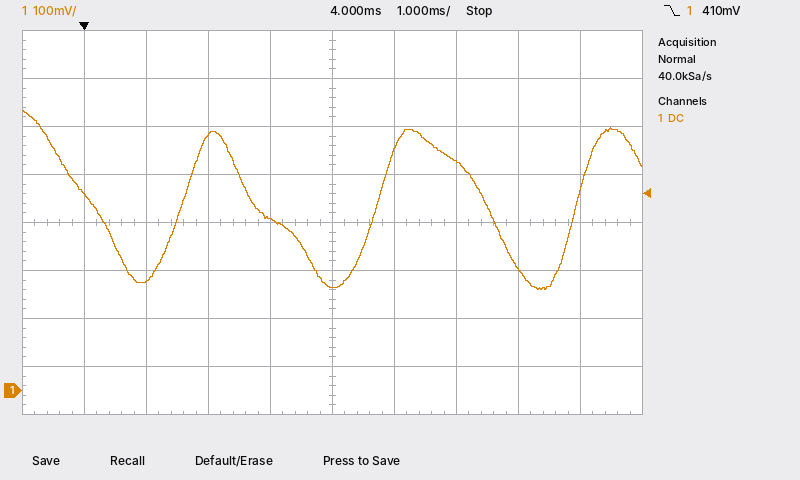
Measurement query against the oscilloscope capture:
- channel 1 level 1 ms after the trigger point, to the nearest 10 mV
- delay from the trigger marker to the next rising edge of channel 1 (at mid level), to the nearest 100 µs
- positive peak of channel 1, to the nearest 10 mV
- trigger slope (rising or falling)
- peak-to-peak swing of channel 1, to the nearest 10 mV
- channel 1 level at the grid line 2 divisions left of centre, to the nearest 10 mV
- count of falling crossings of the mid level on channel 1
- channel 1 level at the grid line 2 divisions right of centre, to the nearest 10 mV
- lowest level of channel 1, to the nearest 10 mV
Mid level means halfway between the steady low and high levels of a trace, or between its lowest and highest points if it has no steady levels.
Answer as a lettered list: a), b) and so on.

a) 230 mV
b) 1.6 ms
c) 580 mV
d) falling
e) 370 mV
f) 530 mV
g) 3
h) 480 mV
i) 210 mV
